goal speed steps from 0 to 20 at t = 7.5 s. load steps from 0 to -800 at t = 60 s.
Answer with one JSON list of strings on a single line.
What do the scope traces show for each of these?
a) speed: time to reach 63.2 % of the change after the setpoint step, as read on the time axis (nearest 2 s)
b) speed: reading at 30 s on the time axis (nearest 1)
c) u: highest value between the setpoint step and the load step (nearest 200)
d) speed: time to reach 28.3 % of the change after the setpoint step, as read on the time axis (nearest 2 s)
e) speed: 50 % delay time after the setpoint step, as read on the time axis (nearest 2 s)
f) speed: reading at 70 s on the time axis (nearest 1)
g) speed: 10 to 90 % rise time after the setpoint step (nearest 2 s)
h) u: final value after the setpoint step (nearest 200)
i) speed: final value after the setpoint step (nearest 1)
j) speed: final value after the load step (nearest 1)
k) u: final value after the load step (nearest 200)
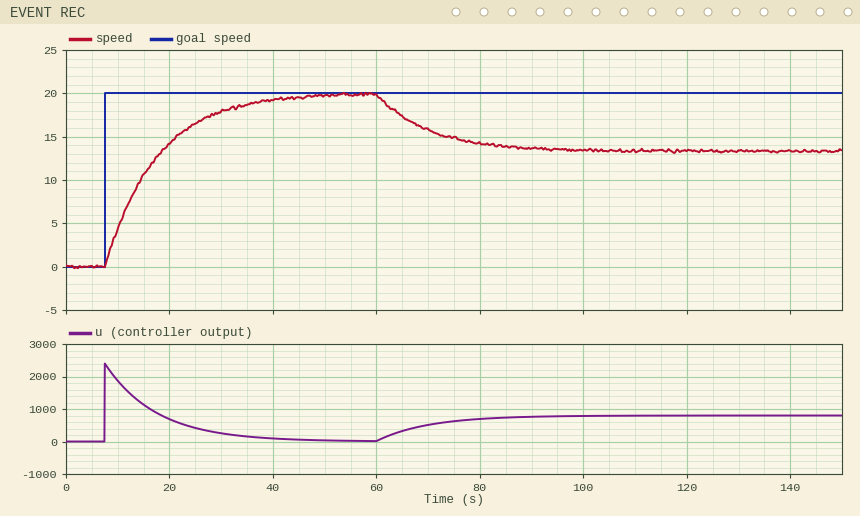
["18 s", "18", "2400", "10 s", "14 s", "16", "22 s", "0", "20", "13", "800"]
